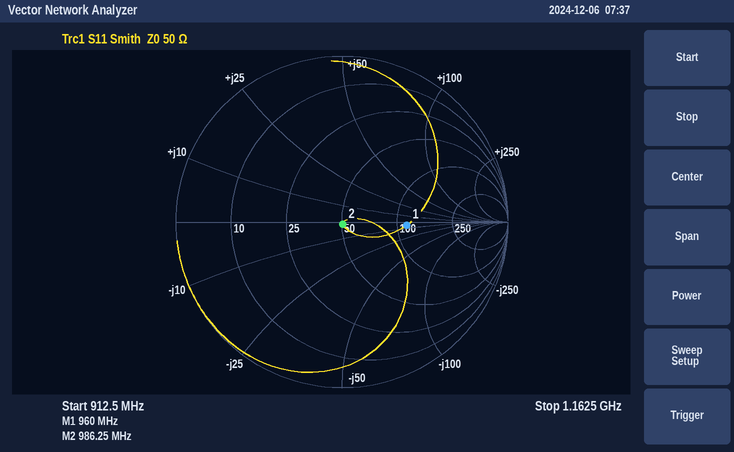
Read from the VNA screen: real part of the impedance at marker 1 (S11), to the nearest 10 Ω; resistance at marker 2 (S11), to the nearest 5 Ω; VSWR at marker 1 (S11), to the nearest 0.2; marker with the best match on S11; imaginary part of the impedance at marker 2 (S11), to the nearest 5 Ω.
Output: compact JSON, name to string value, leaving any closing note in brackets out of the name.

{"real part of the impedance at marker 1 (S11), to the nearest 10 Ω": "110 Ω", "resistance at marker 2 (S11), to the nearest 5 Ω": "50 Ω", "VSWR at marker 1 (S11), to the nearest 0.2": "2.2", "marker with the best match on S11": "marker 2", "imaginary part of the impedance at marker 2 (S11), to the nearest 5 Ω": "0 Ω"}
